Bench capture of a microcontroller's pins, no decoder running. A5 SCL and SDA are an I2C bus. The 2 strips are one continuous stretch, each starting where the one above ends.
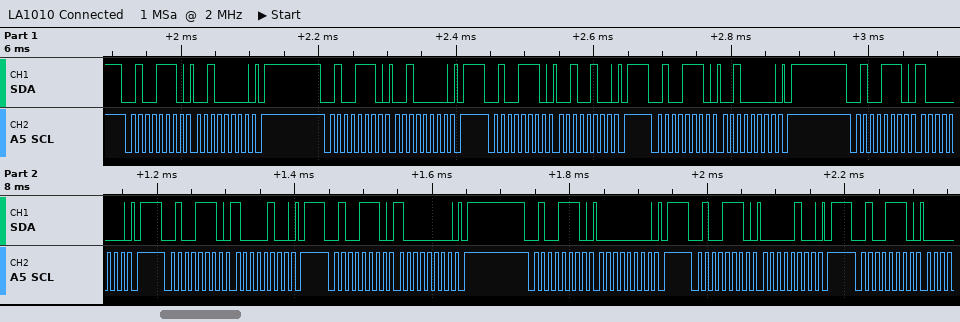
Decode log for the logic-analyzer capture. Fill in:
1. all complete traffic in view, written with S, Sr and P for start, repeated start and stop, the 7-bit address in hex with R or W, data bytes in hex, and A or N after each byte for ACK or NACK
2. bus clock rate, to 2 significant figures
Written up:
S 27W A 20 A P S 27W A 20 A P S 27W A 24 A P S 27W A 20 A P S 27W A 80 A P S 27W A 84 A P S 27W A 80 A P S 27W A 00 A P S 27W A 04 A P S 27W A
100 kHz
